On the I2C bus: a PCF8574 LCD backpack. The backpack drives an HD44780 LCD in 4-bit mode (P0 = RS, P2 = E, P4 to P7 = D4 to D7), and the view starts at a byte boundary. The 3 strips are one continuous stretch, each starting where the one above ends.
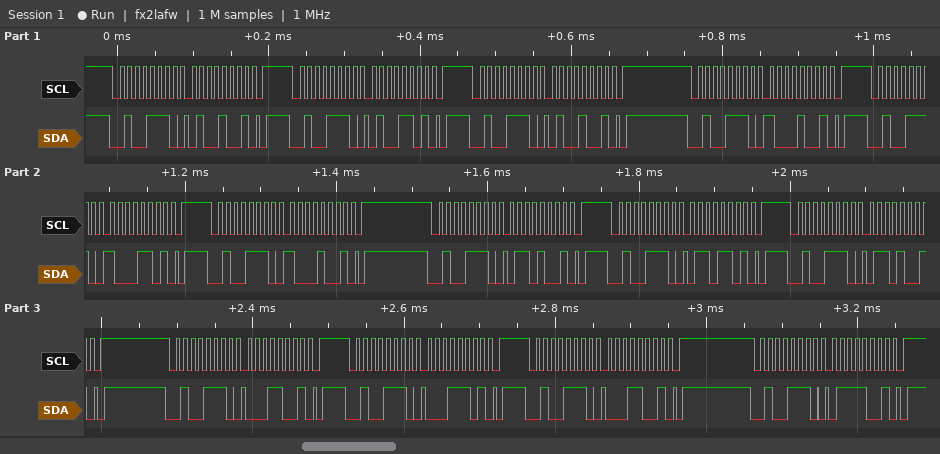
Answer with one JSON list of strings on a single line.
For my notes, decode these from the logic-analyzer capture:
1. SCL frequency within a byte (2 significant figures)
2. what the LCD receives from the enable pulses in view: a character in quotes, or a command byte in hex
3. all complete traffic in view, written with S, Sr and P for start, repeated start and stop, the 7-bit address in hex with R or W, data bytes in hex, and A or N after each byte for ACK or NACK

["100 kHz", "'H' 'a'", "S 27W A 49 A P S 27W A 4D A P S 27W A 49 A P S 27W A 89 A P S 27W A 8D A P S 27W A 89 A P S 27W A 69 A P S 27W A 6D A P S 27W A 69 A P S 27W A 19 A P S 27W A 1D A P S 27W A 19 A P S 27W A 79 A P"]
